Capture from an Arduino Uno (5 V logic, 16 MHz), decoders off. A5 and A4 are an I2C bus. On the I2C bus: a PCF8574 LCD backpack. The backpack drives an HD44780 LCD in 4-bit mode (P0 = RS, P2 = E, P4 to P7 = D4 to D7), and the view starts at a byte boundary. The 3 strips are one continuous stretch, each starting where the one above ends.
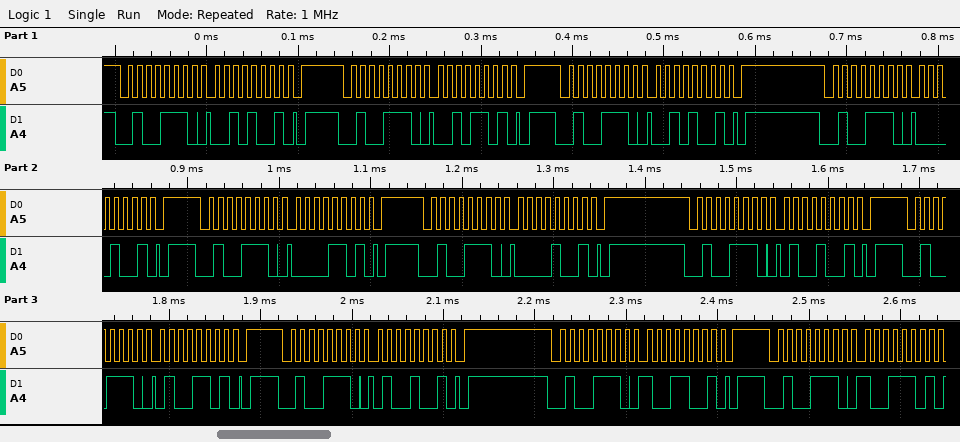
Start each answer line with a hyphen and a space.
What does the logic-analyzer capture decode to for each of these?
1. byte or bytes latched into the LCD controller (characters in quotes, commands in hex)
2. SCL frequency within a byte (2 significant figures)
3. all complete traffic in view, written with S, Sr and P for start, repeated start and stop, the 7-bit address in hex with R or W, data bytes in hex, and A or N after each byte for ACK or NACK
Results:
- ' '
- 100 kHz
- S 27W A 29 A P S 27W A 2D A P S 27W A 29 A P S 27W A 09 A P S 27W A 0D A P S 27W A 09 A P S 27W A 49 A P S 27W A 4D A P S 27W A 49 A P S 27W A 99 A P S 27W A 9D A
